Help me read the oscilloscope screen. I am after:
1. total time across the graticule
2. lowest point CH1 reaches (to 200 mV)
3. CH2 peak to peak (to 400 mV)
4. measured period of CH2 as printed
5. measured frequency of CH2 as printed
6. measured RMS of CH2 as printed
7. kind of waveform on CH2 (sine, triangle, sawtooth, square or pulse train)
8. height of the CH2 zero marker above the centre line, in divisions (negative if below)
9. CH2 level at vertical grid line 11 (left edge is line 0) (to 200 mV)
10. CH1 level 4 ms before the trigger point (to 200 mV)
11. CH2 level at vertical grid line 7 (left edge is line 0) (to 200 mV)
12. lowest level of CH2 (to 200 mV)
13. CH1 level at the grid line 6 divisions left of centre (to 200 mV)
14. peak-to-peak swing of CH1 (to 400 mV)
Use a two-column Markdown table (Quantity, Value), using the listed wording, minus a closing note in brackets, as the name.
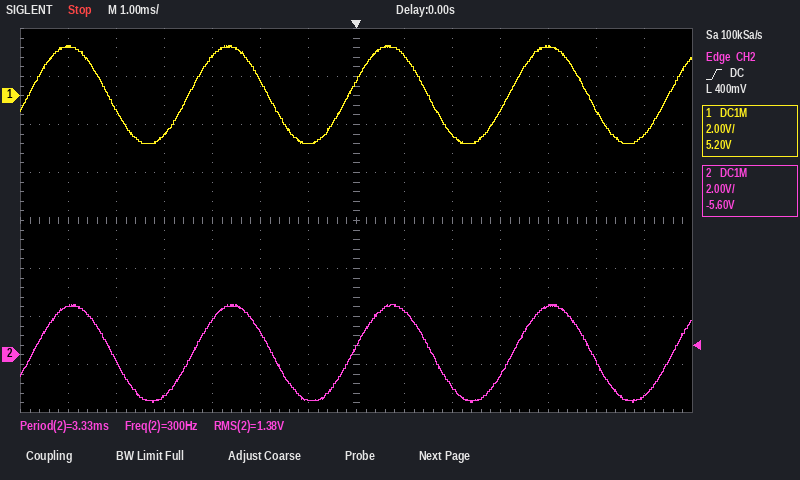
| Quantity | Value |
|---|---|
| total time across the graticule | 14 ms |
| lowest point CH1 reaches | -2.0 V |
| CH2 peak to peak | 4.0 V |
| measured period of CH2 as printed | 3.33 ms |
| measured frequency of CH2 as printed | 300 Hz |
| measured RMS of CH2 as printed | 1.38 V |
| kind of waveform on CH2 | sine |
| height of the CH2 zero marker above the centre line, in divisions | -2.8 div |
| CH2 level at vertical grid line 11 (left edge is line 0) | 2.0 V |
| CH1 level 4 ms before the trigger point | -1.6 V |
| CH2 level at vertical grid line 7 (left edge is line 0) | 400 mV |
| lowest level of CH2 | -2.0 V |
| CH1 level at the grid line 6 divisions left of centre | 2.0 V |
| peak-to-peak swing of CH1 | 4.0 V |
